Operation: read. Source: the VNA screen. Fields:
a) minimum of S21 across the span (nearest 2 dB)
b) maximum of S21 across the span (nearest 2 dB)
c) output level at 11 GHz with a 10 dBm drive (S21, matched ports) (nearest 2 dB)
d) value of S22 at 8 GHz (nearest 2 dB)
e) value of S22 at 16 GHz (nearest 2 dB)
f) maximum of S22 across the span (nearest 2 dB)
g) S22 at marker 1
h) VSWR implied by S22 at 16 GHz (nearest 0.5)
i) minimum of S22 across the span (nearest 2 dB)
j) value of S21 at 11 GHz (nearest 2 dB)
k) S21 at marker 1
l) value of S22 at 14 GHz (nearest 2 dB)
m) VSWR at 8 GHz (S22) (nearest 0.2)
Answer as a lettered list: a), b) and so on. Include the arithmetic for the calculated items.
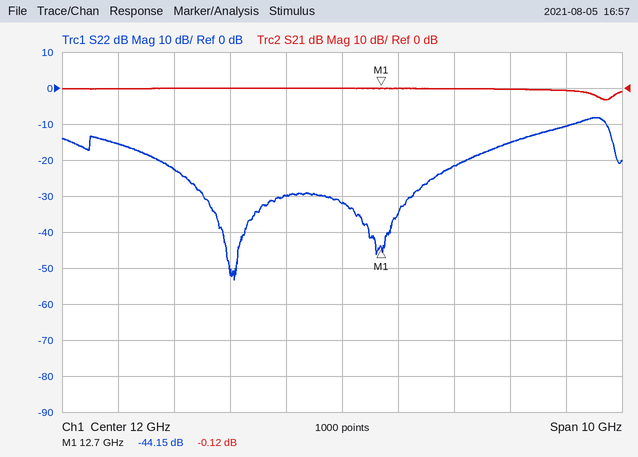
a) -4 dB
b) 0 dB
c) 10 dBm + (0 dB) = 10 dBm
d) -16 dB
e) -10 dB
f) -8 dB
g) -44.15 dB
h) |Γ| = 10^(-10/20) = 0.3162; VSWR = (1 + 0.3162)/(1 − 0.3162) ≈ 1.92, so 2.0 to the nearest 0.5
i) -54 dB
j) 0 dB
k) -0.12 dB
l) -22 dB
m) |Γ| = 10^(-16/20) = 0.1585; VSWR = (1 + 0.1585)/(1 − 0.1585) ≈ 1.4
